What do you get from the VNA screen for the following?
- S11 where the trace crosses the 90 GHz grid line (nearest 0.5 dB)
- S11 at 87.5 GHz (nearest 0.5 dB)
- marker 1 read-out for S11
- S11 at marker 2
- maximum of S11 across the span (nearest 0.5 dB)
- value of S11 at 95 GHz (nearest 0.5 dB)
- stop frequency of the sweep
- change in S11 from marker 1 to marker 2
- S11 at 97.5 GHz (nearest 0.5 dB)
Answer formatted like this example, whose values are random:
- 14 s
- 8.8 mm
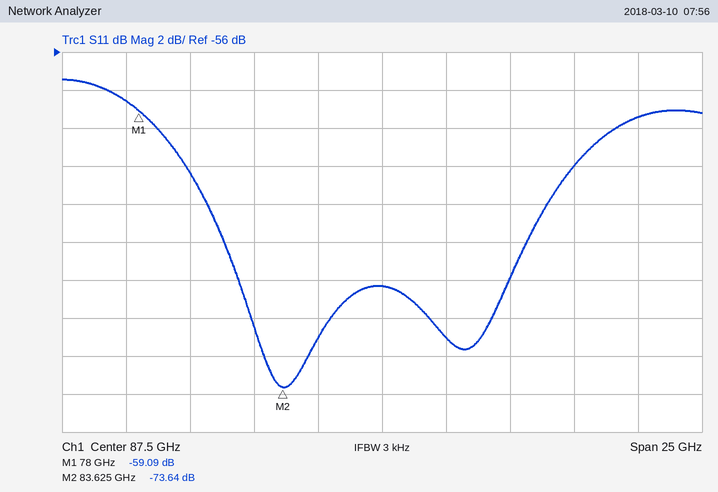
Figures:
- -71.0 dB
- -68.5 dB
- -59.09 dB
- -73.64 dB
- -57.5 dB
- -62.0 dB
- 100 GHz
- -14.55 dB
- -59.5 dB
